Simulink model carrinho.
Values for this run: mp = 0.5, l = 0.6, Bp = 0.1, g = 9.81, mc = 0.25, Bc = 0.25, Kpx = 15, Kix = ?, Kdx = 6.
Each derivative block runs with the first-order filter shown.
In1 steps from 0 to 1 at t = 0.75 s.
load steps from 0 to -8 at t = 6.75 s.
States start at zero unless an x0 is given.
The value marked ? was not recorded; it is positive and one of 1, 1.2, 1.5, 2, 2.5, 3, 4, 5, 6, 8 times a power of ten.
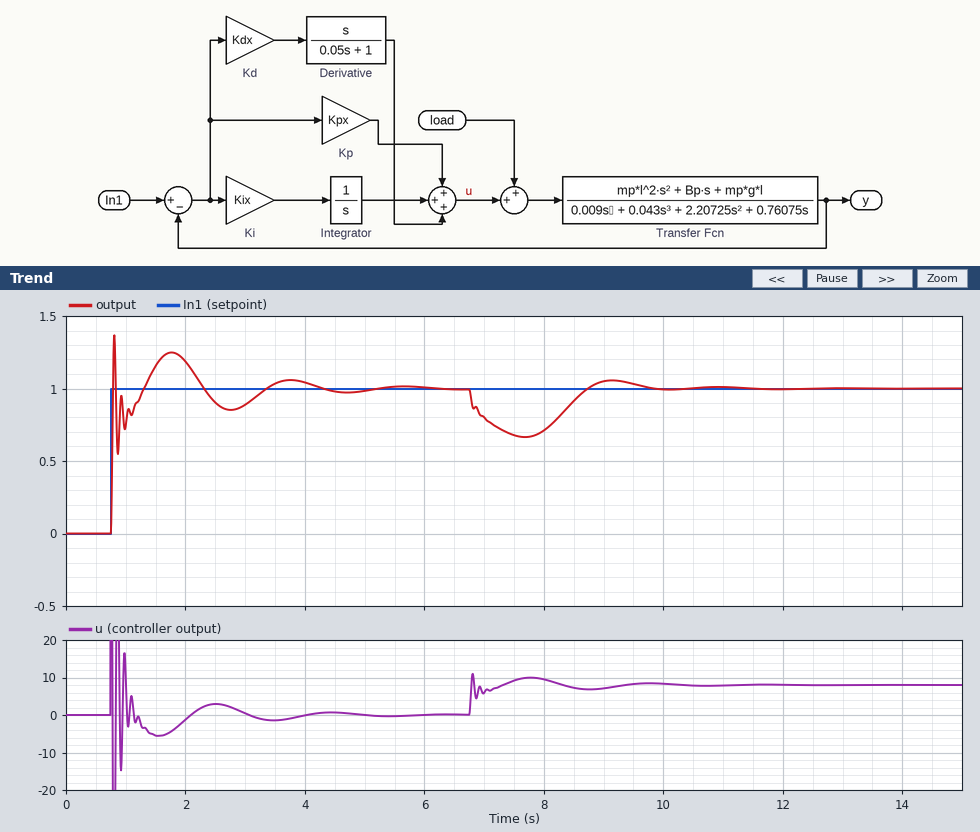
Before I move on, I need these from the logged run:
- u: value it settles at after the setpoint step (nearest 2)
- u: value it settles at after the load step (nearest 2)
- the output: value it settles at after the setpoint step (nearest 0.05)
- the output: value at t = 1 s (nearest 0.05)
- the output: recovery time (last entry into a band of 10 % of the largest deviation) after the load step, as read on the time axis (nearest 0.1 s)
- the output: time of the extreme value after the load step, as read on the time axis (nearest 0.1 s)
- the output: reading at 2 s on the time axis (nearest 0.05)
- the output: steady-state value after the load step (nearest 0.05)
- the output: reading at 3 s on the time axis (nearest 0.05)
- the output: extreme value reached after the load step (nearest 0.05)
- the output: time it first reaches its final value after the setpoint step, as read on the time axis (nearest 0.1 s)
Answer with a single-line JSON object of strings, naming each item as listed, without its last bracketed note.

{"u: value it settles at after the setpoint step": "0", "u: value it settles at after the load step": "8", "the output: value it settles at after the setpoint step": "1.00", "the output: value at t = 1 s": "0.75", "the output: recovery time (last entry into a band of 10 % of the largest deviation) after the load step, as read on the time axis": "9.5 s", "the output: time of the extreme value after the load step, as read on the time axis": "7.7 s", "the output: reading at 2 s on the time axis": "1.20", "the output: steady-state value after the load step": "1.00", "the output: reading at 3 s on the time axis": "0.90", "the output: extreme value reached after the load step": "0.65", "the output: time it first reaches its final value after the setpoint step, as read on the time axis": "0.8 s"}
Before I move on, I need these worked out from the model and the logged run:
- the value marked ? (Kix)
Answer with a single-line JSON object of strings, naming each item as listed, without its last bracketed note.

{"the value marked ?": "20"}
